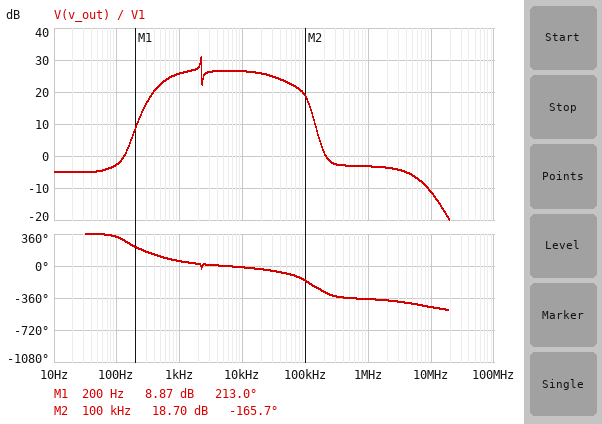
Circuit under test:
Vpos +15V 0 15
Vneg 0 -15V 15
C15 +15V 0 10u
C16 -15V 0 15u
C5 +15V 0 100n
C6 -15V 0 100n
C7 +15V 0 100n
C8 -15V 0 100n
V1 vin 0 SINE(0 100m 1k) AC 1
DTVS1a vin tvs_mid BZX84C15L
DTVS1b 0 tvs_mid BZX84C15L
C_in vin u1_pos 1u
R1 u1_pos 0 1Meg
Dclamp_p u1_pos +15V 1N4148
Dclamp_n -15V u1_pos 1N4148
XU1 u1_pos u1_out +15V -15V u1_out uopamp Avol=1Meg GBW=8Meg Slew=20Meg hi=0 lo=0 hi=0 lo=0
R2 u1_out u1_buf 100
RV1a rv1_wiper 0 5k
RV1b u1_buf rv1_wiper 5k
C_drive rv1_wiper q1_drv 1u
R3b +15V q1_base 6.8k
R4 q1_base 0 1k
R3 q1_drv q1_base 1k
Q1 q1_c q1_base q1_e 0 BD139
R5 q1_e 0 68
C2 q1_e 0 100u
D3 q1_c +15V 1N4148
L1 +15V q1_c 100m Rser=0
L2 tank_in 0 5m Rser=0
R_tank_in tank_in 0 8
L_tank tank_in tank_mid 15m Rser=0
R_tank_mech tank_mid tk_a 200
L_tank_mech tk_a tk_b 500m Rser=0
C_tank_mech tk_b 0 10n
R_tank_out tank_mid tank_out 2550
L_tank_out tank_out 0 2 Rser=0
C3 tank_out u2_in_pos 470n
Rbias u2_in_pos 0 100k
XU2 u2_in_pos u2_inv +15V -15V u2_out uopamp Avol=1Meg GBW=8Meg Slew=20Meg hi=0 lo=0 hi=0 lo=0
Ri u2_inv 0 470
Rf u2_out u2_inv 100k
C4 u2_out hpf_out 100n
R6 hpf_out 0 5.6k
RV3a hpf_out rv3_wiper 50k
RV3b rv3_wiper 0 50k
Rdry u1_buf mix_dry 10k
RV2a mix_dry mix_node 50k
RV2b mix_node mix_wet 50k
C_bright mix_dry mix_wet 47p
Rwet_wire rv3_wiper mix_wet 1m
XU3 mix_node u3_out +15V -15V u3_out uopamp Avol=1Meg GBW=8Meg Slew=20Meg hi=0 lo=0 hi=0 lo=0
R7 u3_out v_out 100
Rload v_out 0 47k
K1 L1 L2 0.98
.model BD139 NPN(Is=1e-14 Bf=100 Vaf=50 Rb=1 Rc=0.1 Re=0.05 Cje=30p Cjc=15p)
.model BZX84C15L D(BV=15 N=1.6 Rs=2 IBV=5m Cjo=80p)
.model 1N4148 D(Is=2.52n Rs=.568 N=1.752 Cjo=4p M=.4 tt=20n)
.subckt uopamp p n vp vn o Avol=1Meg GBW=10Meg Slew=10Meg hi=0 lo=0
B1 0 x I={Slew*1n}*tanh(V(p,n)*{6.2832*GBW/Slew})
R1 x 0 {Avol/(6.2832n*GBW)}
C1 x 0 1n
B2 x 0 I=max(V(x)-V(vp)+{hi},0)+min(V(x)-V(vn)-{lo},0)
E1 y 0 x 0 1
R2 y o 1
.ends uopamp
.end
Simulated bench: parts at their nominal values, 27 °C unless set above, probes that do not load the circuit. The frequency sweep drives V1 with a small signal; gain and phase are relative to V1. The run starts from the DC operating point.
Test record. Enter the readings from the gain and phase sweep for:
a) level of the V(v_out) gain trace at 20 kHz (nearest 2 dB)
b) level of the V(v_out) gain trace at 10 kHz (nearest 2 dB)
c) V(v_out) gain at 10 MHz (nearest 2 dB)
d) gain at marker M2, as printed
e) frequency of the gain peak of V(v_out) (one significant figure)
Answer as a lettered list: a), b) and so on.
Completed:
a) 26 dB
b) 26 dB
c) -12 dB
d) 18.70 dB
e) 2 kHz
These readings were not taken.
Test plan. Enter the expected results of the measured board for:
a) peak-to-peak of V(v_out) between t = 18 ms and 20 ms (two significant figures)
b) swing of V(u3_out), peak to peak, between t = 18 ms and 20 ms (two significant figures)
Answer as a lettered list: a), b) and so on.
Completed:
a) 3.9 V
b) 3.9 V
